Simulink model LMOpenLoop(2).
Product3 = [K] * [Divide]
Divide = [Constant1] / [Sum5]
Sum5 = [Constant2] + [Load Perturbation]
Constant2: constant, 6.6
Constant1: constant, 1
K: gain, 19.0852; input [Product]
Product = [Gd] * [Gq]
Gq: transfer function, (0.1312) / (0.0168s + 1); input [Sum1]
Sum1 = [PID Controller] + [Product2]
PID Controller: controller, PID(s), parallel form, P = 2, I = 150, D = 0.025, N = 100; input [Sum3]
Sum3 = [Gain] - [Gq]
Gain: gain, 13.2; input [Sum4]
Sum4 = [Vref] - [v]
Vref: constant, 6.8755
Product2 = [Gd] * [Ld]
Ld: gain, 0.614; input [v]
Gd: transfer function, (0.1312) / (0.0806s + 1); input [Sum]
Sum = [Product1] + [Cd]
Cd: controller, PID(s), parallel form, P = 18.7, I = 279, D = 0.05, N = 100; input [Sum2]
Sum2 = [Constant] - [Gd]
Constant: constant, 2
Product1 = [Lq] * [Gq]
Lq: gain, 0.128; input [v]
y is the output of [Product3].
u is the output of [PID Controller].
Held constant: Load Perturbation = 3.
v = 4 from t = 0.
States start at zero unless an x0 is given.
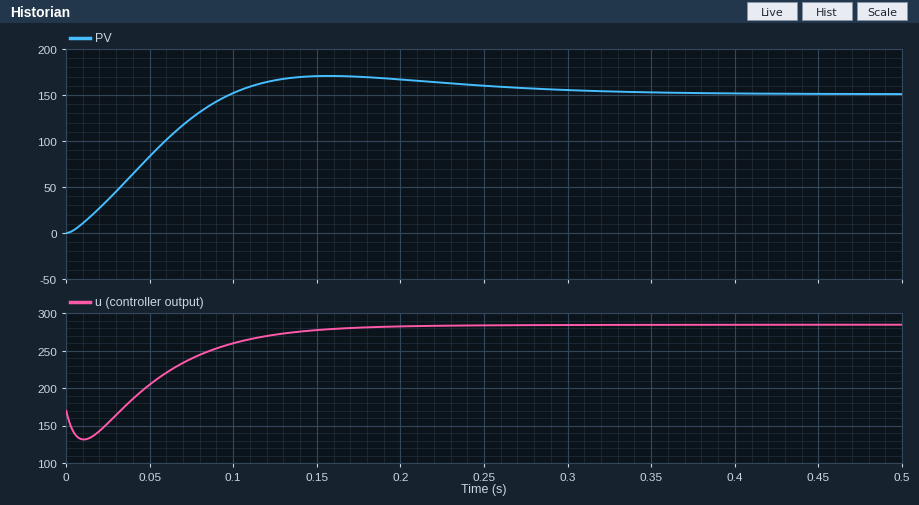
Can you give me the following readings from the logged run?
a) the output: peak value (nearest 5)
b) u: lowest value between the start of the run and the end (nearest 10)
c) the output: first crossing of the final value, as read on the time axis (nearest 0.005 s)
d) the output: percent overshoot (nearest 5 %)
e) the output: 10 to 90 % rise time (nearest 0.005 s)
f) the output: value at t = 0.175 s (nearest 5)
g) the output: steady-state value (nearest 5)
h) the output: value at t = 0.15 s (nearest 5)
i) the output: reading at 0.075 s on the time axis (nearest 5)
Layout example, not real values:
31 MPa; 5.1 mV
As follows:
170; 130; 0.100 s; 15 %; 0.070 s; 170; 150; 170; 125
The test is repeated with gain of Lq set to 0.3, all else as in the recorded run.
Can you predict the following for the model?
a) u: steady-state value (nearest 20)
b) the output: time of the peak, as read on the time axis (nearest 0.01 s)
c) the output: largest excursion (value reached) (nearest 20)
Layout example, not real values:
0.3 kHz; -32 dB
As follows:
280; 0.14 s; 200
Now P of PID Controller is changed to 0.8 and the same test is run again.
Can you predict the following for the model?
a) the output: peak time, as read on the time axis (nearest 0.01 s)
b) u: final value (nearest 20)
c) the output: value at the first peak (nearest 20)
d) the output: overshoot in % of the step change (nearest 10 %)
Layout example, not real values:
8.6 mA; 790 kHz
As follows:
0.15 s; 280; 180; 20 %
